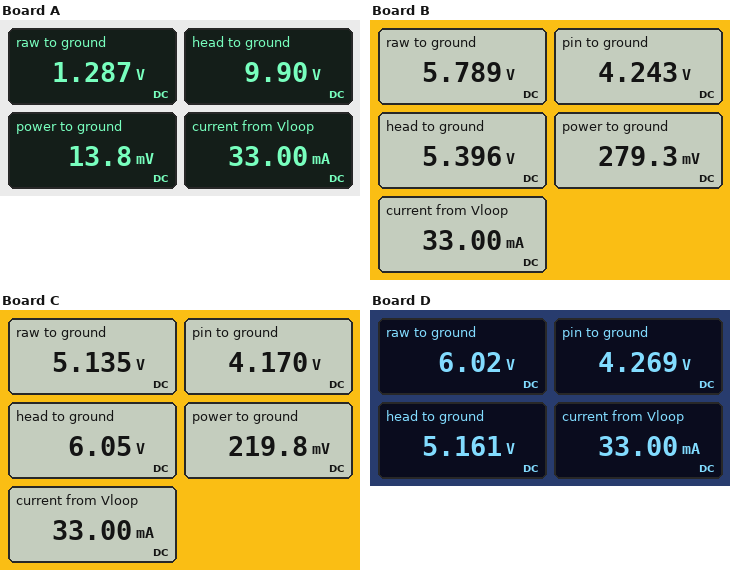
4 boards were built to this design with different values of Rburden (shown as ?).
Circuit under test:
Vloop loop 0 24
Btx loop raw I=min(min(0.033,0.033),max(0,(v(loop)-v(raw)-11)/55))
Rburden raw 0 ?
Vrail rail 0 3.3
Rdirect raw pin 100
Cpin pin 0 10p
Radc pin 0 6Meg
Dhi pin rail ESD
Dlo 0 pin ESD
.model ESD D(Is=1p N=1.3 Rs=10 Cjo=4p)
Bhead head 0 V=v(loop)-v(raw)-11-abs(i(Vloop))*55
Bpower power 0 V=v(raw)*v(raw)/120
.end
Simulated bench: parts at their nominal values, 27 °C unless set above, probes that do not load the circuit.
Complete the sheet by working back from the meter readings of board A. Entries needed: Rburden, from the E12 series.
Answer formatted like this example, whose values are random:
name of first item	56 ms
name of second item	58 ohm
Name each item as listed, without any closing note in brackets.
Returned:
Rburden, from the E12 series	39 Ω
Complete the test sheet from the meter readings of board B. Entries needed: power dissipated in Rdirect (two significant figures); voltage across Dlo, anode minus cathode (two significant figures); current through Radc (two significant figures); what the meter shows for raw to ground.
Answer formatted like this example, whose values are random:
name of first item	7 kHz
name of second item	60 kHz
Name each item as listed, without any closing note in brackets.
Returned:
power dissipated in Rdirect	24 mW
voltage across Dlo, anode minus cathode	-4.2 V
current through Radc	710 nA
what the meter shows for raw to ground	5.789 V
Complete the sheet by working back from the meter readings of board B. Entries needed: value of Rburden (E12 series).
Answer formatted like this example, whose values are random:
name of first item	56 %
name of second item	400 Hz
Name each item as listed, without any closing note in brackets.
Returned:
value of Rburden	330 Ω
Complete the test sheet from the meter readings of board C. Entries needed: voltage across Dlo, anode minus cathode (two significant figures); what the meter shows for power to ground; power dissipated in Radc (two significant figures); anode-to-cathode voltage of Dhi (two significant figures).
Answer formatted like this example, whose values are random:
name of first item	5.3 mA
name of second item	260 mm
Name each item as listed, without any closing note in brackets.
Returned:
voltage across Dlo, anode minus cathode	-4.2 V
what the meter shows for power to ground	219.8 mV
power dissipated in Radc	2.9 µW
anode-to-cathode voltage of Dhi	870 mV
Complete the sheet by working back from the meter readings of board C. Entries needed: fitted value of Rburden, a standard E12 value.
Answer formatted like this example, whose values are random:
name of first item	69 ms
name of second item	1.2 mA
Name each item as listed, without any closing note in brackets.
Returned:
fitted value of Rburden, a standard E12 value	220 Ω
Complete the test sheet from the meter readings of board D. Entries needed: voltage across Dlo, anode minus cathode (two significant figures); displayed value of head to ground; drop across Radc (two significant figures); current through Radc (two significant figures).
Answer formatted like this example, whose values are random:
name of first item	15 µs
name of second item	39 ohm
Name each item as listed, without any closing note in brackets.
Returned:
voltage across Dlo, anode minus cathode	-4.3 V
displayed value of head to ground	5.161 V
drop across Radc	4.3 V
current through Radc	710 nA
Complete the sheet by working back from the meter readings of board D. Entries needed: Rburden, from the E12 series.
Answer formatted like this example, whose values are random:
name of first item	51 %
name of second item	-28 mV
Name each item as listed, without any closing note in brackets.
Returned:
Rburden, from the E12 series	390 Ω
